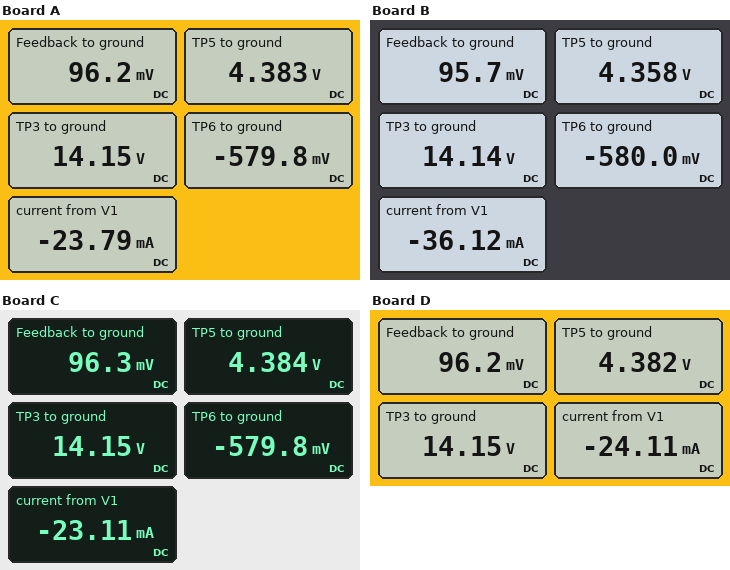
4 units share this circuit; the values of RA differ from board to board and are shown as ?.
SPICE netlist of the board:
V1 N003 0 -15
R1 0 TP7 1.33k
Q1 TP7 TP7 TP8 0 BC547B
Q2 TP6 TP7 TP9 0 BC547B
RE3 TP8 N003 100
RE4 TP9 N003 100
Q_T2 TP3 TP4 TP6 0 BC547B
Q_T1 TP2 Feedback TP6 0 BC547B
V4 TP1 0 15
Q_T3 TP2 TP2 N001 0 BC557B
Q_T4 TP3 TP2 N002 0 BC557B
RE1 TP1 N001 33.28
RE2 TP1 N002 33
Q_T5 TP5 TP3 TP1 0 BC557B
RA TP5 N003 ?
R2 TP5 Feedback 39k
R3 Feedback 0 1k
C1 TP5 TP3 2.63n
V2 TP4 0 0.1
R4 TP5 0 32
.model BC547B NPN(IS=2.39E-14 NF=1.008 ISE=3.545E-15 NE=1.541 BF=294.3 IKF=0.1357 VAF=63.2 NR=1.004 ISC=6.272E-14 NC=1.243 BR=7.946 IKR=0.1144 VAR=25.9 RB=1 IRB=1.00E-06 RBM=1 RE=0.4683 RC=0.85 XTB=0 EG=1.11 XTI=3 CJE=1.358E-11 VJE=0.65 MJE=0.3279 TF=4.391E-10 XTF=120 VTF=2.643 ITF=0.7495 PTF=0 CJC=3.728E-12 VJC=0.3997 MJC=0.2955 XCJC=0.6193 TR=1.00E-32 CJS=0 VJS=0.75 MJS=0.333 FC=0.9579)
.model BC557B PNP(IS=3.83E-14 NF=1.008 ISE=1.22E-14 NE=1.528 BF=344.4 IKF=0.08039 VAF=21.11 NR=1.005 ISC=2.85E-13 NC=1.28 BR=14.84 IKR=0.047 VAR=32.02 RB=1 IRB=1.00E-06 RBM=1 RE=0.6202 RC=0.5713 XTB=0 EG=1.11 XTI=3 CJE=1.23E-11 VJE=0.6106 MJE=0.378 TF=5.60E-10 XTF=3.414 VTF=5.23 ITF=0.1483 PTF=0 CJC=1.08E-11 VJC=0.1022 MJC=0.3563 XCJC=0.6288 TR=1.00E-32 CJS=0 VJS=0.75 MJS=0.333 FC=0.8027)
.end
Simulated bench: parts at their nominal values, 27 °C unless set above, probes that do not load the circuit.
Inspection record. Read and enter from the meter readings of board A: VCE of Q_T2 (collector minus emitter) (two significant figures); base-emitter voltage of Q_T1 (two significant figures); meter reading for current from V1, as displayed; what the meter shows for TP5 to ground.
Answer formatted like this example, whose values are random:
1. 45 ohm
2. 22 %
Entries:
1. 15 V
2. 680 mV
3. -23.79 mA
4. 4.383 V
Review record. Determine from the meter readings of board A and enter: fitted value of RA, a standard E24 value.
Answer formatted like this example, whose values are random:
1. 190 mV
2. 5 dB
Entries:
1. 5.1 kΩ
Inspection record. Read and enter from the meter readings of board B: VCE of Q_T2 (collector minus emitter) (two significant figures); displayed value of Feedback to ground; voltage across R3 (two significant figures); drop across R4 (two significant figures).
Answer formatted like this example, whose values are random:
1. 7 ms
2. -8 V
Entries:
1. 15 V
2. 95.7 mV
3. 96 mV
4. 4.4 V
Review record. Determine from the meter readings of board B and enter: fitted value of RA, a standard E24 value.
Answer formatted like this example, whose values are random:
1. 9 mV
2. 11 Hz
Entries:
1. 1.2 kΩ
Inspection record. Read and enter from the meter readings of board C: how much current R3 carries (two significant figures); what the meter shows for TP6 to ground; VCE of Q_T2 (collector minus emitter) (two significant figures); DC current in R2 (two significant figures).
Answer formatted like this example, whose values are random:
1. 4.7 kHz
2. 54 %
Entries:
1. 96 µA
2. -579.8 mV
3. 15 V
4. 110 µA
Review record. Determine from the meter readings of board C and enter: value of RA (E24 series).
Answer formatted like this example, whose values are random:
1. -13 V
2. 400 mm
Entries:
1. 6.2 kΩ
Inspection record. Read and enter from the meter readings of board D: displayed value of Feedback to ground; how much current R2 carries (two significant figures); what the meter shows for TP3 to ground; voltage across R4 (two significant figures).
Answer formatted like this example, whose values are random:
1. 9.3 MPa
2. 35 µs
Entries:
1. 96.2 mV
2. 110 µA
3. 14.15 V
4. 4.4 V
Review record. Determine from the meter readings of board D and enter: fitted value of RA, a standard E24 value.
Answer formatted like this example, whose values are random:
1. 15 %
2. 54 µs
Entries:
1. 4.7 kΩ
